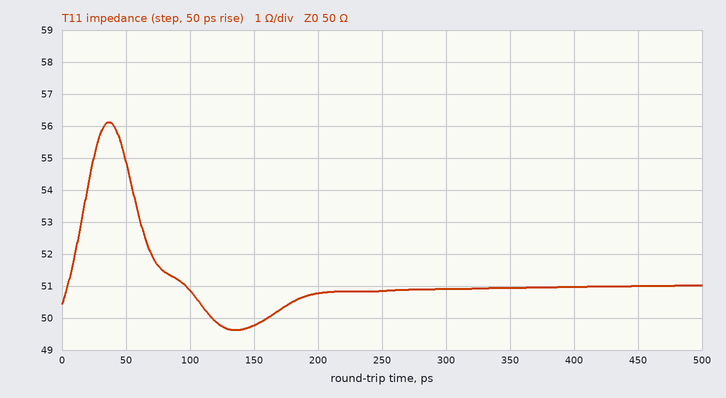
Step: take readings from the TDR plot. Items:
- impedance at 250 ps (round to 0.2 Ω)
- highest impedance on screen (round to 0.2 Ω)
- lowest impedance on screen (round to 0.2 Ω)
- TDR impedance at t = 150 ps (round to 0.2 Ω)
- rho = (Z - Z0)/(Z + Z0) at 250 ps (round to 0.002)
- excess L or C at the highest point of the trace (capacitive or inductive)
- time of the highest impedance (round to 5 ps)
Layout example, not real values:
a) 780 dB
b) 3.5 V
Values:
a) 50.8 Ω
b) 56.2 Ω
c) 49.6 Ω
d) 49.8 Ω
e) +0.008
f) inductive
g) 35 ps
